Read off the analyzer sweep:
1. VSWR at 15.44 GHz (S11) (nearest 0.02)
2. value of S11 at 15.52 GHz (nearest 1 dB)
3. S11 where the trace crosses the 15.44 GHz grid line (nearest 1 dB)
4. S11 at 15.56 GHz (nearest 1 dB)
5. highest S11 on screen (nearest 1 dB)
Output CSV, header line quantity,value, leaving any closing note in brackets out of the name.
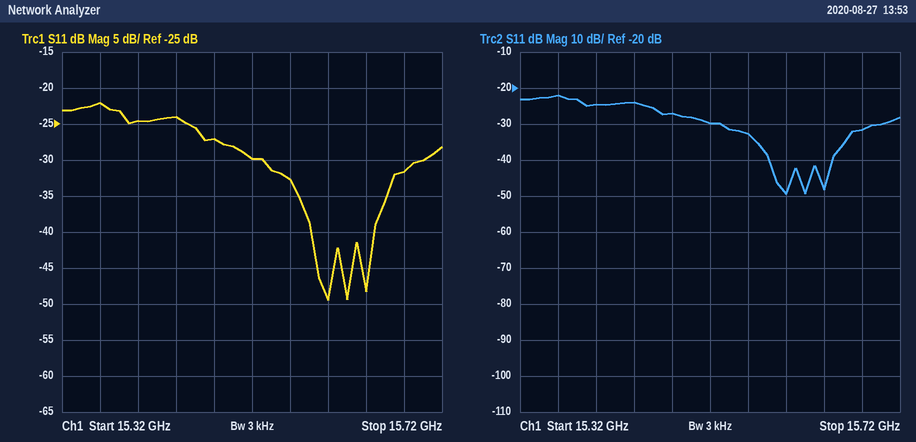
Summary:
quantity,value
VSWR at 15.44 GHz (S11),1.14
value of S11 at 15.52 GHz,-30 dB
S11 where the trace crosses the 15.44 GHz grid line,-24 dB
S11 at 15.56 GHz,-33 dB
highest S11 on screen,-22 dB
